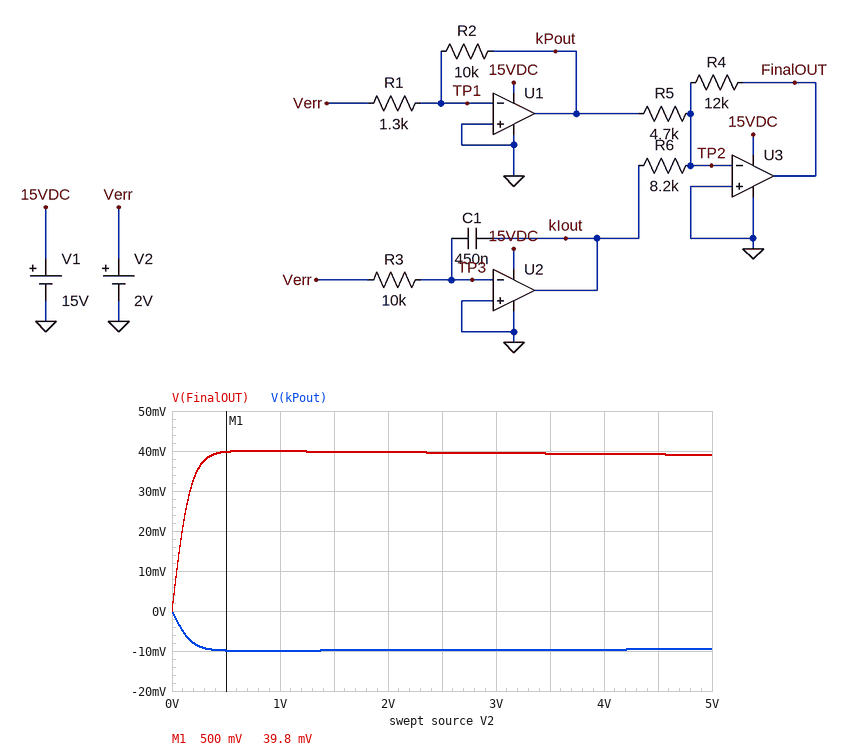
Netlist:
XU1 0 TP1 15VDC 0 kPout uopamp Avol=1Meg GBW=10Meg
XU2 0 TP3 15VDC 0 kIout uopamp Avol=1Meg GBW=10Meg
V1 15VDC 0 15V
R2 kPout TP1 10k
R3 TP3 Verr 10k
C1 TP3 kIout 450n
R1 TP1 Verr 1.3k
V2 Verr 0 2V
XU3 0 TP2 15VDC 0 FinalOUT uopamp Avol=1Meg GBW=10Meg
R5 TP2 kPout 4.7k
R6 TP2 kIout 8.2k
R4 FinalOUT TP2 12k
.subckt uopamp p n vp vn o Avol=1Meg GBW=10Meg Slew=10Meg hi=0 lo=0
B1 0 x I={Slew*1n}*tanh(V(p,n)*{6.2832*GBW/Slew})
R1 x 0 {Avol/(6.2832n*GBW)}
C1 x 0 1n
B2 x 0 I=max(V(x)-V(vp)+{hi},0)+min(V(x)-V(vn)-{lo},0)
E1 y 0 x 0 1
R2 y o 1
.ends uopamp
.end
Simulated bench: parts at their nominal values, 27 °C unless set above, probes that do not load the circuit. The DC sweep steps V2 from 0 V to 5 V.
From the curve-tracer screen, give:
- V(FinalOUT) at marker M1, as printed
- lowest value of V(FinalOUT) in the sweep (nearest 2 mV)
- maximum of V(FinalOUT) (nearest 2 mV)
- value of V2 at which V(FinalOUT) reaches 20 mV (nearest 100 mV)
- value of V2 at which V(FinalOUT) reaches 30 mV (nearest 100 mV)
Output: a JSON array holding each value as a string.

["39.8 mV", "0 V", "40 mV", "100 mV", "200 mV"]
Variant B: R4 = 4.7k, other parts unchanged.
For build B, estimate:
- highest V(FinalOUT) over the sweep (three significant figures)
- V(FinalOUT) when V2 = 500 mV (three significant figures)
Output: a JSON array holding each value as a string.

["15.7 mV", "15.6 mV"]
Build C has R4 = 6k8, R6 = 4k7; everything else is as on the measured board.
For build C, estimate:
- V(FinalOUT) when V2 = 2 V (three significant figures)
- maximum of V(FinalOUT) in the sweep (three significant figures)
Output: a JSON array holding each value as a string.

["28.7 mV", "28.8 mV"]
